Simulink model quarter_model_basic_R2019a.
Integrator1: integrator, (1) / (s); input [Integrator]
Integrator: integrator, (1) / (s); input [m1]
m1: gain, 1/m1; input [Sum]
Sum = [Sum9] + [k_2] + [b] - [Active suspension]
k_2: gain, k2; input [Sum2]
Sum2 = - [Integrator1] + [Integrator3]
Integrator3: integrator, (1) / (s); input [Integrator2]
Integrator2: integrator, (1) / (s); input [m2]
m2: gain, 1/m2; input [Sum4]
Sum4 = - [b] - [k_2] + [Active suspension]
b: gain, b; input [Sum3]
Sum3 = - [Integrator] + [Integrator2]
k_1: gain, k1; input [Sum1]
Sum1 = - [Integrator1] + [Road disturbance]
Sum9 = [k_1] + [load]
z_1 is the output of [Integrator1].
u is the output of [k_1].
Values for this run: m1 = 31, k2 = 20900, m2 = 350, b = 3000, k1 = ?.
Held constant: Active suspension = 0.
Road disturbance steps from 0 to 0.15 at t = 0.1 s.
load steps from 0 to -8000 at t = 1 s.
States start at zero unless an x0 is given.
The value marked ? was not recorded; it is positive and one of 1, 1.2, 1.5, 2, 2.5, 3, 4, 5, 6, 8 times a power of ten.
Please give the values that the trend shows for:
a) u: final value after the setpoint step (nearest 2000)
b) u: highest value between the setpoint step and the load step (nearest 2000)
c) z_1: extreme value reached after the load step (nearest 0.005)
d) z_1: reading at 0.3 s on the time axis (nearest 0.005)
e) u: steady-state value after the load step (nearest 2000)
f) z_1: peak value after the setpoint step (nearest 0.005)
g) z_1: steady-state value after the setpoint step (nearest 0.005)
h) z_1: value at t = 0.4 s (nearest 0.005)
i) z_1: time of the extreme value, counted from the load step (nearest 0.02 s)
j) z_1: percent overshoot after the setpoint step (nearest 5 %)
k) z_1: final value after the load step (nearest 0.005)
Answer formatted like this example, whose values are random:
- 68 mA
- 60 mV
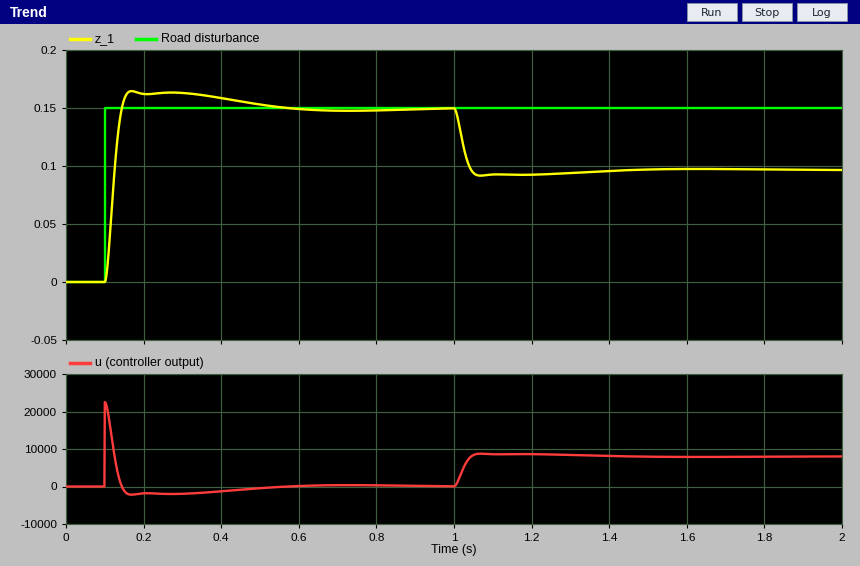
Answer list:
- 0
- 22000
- 0.090
- 0.165
- 8000
- 0.165
- 0.150
- 0.160
- 0.06 s
- 10 %
- 0.095
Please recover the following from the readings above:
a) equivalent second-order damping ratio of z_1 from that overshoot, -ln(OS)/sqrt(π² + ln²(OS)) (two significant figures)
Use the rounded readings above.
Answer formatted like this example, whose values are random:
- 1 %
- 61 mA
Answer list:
- 0.59
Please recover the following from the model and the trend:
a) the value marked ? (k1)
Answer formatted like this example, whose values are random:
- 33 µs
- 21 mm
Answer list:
- 150000
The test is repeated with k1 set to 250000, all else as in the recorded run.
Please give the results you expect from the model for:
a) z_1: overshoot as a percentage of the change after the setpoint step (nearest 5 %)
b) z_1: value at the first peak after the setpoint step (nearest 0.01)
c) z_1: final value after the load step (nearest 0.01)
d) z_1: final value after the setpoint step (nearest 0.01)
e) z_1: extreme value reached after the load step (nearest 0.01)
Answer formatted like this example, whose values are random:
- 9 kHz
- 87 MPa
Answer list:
- 15 %
- 0.17
- 0.12
- 0.15
- 0.11
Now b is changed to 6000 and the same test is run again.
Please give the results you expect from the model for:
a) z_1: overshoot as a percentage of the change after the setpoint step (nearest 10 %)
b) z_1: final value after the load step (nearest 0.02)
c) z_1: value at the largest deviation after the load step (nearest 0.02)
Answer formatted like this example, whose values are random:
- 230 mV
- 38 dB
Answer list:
- 30 %
- 0.10
- 0.08
